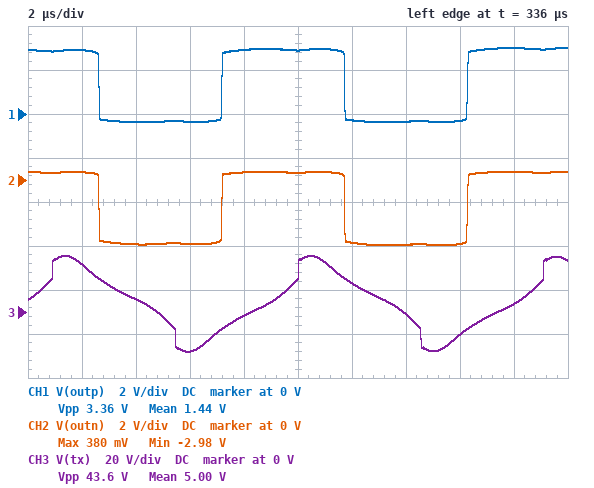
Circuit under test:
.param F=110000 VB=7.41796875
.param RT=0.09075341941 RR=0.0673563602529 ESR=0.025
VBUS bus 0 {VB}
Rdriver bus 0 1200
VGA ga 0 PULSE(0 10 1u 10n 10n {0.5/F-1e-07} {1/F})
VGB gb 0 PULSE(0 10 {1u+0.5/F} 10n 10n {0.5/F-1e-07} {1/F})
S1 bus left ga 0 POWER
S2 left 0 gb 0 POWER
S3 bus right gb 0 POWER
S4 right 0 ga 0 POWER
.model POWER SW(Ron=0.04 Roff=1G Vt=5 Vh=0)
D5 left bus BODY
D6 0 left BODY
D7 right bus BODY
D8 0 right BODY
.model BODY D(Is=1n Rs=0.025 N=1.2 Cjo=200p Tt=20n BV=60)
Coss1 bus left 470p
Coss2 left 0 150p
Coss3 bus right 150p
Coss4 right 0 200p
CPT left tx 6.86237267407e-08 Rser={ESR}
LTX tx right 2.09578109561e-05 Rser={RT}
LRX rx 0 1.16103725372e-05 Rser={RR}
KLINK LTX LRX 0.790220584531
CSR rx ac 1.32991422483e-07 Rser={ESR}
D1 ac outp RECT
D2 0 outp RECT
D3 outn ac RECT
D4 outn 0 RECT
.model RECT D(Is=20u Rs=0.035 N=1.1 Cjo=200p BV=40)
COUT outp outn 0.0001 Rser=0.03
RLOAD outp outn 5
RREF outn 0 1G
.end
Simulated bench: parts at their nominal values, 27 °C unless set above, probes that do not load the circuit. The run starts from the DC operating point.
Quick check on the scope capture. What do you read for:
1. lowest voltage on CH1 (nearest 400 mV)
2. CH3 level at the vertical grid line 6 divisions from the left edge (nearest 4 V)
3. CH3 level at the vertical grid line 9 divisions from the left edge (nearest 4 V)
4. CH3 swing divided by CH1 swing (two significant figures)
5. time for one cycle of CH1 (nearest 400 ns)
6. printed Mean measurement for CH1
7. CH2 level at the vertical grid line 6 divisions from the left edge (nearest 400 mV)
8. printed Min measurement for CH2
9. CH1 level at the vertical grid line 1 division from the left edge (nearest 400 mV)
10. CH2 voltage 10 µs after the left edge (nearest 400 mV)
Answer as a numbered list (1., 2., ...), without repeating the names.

1. -400 mV
2. 12 V
3. 4 V
4. 13
5. 9.2 µs
6. 1.44 V
7. -2.8 V
8. -2.98 V
9. 2.8 V
10. 400 mV
